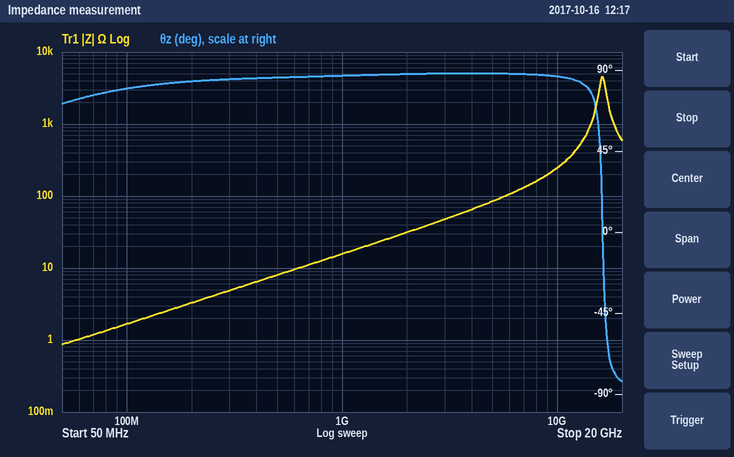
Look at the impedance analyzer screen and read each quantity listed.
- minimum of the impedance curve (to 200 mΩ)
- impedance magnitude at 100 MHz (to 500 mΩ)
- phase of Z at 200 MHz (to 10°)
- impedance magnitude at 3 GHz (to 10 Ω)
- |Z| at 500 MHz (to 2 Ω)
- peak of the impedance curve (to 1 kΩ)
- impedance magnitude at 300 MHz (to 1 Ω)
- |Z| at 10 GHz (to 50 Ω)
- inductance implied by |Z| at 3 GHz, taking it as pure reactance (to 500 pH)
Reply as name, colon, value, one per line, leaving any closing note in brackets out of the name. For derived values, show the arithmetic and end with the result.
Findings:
minimum of the impedance curve: 800 mΩ
impedance magnitude at 100 MHz: 1.5 Ω
phase of Z at 200 MHz: 80°
impedance magnitude at 3 GHz: 50 Ω
|Z| at 500 MHz: 8 Ω
peak of the impedance curve: 5 kΩ
impedance magnitude at 300 MHz: 5 Ω
|Z| at 10 GHz: 250 Ω
inductance implied by |Z| at 3 GHz, taking it as pure reactance: L = 50 Ω/(2π × 3 GHz) ≈ 2.65 nH, so 2.5 nH to the nearest 500 pH
